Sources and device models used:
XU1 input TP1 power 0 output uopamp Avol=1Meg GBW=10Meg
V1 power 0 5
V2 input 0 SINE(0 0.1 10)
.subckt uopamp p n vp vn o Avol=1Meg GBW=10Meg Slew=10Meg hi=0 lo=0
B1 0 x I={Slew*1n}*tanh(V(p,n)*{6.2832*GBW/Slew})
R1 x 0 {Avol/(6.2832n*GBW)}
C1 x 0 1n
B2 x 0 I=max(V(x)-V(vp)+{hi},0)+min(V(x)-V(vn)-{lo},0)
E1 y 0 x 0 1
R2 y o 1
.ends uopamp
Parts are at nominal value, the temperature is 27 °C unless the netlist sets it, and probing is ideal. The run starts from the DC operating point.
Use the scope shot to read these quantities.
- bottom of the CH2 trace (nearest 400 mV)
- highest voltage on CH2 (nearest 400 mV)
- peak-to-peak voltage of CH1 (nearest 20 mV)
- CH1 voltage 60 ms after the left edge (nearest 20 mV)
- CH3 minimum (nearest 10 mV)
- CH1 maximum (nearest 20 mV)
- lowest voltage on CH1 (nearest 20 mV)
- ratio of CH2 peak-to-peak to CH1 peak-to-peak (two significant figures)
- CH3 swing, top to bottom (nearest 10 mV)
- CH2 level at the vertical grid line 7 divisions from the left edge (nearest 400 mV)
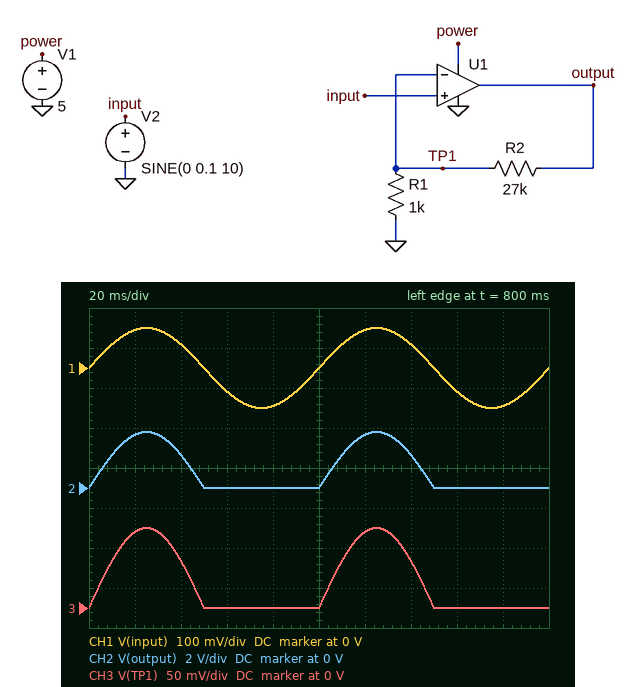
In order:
0 V
2.8 V
200 mV
-60 mV
0 V
100 mV
-100 mV
14
100 mV
1.6 V
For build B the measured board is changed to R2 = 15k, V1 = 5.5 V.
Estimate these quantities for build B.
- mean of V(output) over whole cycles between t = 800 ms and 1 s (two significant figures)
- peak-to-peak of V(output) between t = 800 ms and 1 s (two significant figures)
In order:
510 mV
1.6 V
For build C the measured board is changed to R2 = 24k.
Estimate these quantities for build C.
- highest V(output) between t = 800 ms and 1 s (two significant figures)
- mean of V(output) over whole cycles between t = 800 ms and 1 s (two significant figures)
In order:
2.5 V
790 mV
